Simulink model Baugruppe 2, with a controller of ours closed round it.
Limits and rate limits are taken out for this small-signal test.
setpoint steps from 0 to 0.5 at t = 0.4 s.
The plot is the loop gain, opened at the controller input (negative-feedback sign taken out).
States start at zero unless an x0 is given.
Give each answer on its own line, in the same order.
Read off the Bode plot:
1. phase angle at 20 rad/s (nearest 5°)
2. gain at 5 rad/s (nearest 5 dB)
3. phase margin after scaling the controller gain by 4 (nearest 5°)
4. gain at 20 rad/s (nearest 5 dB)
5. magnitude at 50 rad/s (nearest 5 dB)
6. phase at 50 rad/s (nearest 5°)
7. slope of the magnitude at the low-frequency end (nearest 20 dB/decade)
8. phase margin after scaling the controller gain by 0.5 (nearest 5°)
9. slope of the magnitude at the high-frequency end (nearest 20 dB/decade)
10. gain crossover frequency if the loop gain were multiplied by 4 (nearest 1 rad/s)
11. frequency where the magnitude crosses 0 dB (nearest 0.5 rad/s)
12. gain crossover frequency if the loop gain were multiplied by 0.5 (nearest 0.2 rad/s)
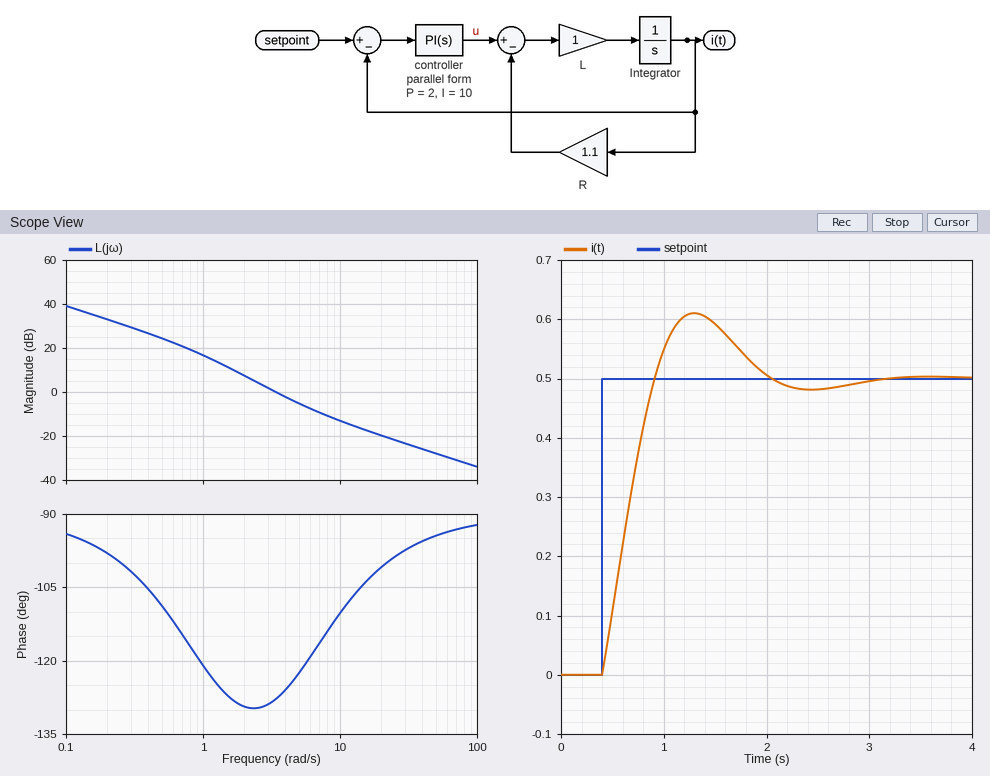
-100°
-5 dB
70°
-20 dB
-30 dB
-95°
-20 dB/decade
50°
-20 dB/decade
9 rad/s
3.5 rad/s
2.2 rad/s
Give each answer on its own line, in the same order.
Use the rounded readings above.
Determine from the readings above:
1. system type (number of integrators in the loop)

1
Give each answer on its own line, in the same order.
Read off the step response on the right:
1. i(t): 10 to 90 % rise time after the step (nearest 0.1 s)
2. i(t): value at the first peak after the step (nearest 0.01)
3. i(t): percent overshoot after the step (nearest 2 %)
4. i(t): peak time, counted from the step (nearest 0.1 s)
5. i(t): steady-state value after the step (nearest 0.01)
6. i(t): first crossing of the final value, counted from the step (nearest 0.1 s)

0.4 s
0.61
22 %
0.9 s
0.50
0.5 s
